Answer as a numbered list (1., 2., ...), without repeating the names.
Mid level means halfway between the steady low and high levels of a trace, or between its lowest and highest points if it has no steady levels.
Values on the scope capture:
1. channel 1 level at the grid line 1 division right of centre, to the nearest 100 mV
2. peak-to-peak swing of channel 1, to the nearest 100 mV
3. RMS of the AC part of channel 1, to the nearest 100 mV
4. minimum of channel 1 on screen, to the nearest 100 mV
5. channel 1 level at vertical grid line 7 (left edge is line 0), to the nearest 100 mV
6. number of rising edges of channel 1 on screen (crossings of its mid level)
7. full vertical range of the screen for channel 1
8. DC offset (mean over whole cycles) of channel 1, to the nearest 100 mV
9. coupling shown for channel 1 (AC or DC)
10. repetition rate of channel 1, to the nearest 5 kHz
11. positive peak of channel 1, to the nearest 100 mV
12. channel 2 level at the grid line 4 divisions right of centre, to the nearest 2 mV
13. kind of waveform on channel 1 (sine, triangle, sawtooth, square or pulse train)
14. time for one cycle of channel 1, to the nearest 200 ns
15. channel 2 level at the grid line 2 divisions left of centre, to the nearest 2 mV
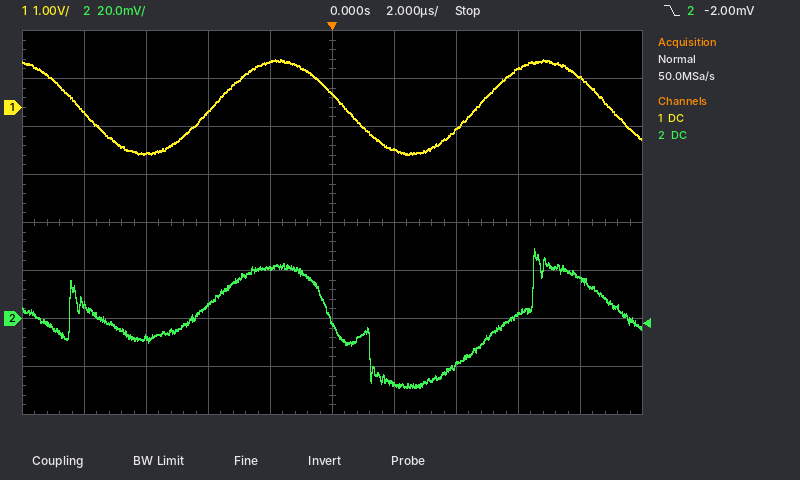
1. -900 mV
2. 2.0 V
3. 700 mV
4. -1.0 V
5. -500 mV
6. 2
7. 8 V
8. 0.0 V
9. DC
10. 115 kHz
11. 1.0 V
12. 16 mV
13. sine
14. 8.6 µs
15. 6 mV
